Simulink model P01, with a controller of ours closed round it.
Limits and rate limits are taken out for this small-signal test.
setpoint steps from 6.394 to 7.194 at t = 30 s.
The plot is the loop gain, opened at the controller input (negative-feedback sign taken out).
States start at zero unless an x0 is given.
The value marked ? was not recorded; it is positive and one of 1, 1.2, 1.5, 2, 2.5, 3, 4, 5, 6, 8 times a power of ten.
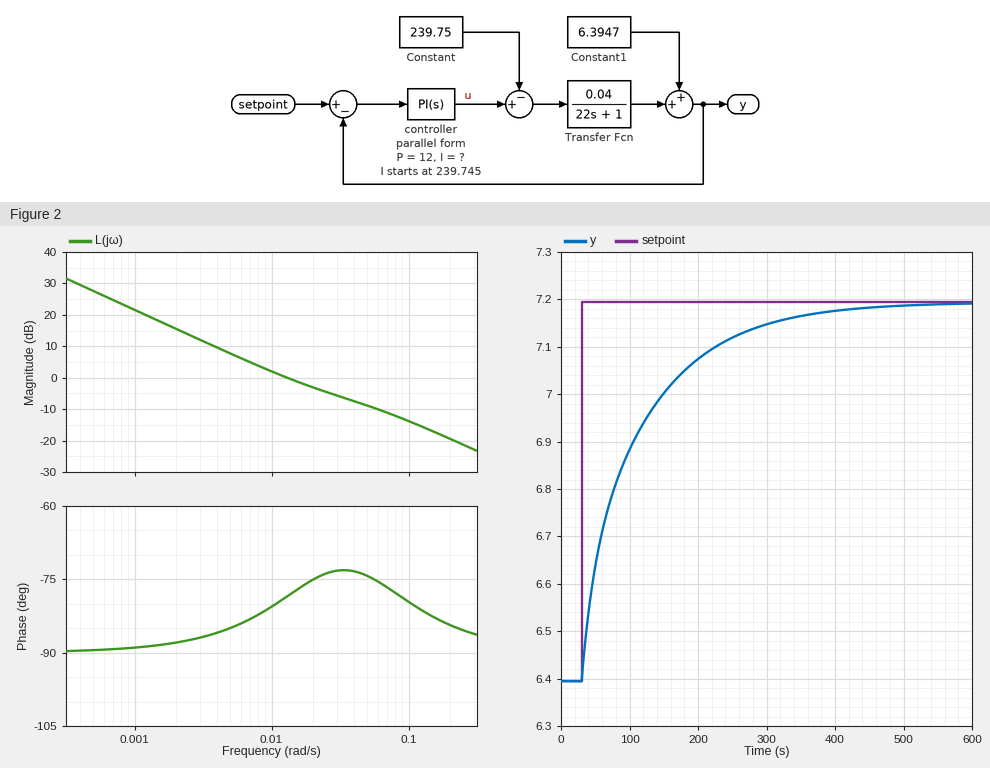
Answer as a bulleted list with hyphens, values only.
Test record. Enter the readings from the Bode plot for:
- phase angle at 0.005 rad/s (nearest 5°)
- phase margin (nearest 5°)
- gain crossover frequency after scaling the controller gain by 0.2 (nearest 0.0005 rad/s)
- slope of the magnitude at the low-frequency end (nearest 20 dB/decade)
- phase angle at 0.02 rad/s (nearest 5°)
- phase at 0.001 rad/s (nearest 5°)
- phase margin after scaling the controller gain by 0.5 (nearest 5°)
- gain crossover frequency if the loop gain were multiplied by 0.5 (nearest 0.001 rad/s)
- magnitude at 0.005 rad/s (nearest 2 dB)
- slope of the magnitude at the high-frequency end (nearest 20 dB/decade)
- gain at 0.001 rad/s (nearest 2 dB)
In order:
- -85°
- 100°
- 0.0025 rad/s
- -20 dB/decade
- -75°
- -90°
- 95°
- 0.006 rad/s
- 8 dB
- -20 dB/decade
- 22 dB
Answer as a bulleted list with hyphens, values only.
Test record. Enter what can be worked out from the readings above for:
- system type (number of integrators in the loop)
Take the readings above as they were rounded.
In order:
- 1
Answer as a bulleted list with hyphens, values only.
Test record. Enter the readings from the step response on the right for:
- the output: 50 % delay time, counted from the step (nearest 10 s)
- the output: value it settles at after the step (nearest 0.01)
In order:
- 50 s
- 7.19
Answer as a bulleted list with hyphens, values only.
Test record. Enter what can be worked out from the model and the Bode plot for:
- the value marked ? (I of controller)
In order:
- 0.3
